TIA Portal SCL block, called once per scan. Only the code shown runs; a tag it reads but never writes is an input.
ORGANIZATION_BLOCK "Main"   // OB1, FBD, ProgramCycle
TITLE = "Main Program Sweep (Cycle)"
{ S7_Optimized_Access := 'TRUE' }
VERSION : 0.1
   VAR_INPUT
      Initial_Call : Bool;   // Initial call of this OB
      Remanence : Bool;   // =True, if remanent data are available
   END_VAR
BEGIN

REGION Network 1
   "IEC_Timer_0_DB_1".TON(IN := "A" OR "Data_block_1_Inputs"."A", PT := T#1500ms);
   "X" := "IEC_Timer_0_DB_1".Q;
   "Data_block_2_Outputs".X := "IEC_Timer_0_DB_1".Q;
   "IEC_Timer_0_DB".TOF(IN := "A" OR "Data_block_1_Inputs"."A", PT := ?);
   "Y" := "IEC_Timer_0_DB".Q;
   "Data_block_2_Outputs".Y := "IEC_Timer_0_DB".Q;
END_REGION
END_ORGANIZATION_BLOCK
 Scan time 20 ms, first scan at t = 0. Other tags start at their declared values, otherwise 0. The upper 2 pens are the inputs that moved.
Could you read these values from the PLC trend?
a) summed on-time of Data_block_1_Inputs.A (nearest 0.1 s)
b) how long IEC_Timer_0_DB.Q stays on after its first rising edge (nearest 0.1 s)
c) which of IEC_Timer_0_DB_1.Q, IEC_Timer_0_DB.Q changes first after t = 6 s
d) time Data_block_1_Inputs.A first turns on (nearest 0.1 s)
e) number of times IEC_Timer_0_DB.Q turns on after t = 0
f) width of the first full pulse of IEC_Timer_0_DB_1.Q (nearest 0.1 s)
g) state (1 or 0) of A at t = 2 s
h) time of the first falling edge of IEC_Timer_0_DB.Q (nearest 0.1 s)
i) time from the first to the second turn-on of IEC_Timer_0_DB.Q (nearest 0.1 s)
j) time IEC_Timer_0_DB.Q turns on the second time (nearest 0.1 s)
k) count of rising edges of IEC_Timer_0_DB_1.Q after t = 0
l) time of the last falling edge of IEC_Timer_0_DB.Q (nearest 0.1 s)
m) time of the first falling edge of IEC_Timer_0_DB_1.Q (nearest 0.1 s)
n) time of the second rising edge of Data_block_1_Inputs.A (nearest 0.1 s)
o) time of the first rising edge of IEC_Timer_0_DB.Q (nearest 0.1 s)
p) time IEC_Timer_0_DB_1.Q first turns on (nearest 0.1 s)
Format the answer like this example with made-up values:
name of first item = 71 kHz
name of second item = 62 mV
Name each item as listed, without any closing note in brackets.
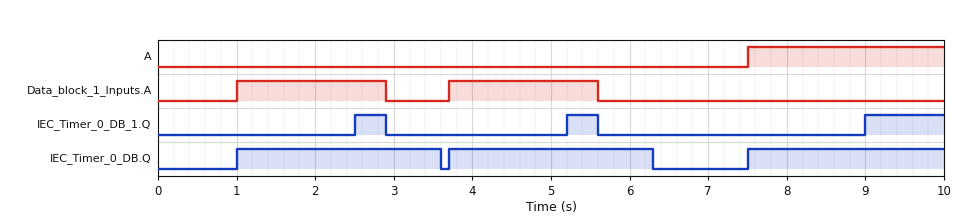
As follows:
summed on-time of Data_block_1_Inputs.A = 3.8 s
how long IEC_Timer_0_DB.Q stays on after its first rising edge = 2.6 s
which of IEC_Timer_0_DB_1.Q, IEC_Timer_0_DB.Q changes first after t = 6 s = IEC_Timer_0_DB.Q
time Data_block_1_Inputs.A first turns on = 1.0 s
number of times IEC_Timer_0_DB.Q turns on after t = 0 = 3
width of the first full pulse of IEC_Timer_0_DB_1.Q = 0.4 s
state (1 or 0) of A at t = 2 s = 0
time of the first falling edge of IEC_Timer_0_DB.Q = 3.6 s
time from the first to the second turn-on of IEC_Timer_0_DB.Q = 2.7 s
time IEC_Timer_0_DB.Q turns on the second time = 3.7 s
count of rising edges of IEC_Timer_0_DB_1.Q after t = 0 = 3
time of the last falling edge of IEC_Timer_0_DB.Q = 6.3 s
time of the first falling edge of IEC_Timer_0_DB_1.Q = 2.9 s
time of the second rising edge of Data_block_1_Inputs.A = 3.7 s
time of the first rising edge of IEC_Timer_0_DB.Q = 1.0 s
time IEC_Timer_0_DB_1.Q first turns on = 2.5 s
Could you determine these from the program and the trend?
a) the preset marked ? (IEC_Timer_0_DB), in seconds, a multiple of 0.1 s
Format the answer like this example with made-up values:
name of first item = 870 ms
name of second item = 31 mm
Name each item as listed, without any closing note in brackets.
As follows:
the preset marked ? (IEC_Timer_0_DB), in seconds, a multiple of 0.1 s = 0.7 s
